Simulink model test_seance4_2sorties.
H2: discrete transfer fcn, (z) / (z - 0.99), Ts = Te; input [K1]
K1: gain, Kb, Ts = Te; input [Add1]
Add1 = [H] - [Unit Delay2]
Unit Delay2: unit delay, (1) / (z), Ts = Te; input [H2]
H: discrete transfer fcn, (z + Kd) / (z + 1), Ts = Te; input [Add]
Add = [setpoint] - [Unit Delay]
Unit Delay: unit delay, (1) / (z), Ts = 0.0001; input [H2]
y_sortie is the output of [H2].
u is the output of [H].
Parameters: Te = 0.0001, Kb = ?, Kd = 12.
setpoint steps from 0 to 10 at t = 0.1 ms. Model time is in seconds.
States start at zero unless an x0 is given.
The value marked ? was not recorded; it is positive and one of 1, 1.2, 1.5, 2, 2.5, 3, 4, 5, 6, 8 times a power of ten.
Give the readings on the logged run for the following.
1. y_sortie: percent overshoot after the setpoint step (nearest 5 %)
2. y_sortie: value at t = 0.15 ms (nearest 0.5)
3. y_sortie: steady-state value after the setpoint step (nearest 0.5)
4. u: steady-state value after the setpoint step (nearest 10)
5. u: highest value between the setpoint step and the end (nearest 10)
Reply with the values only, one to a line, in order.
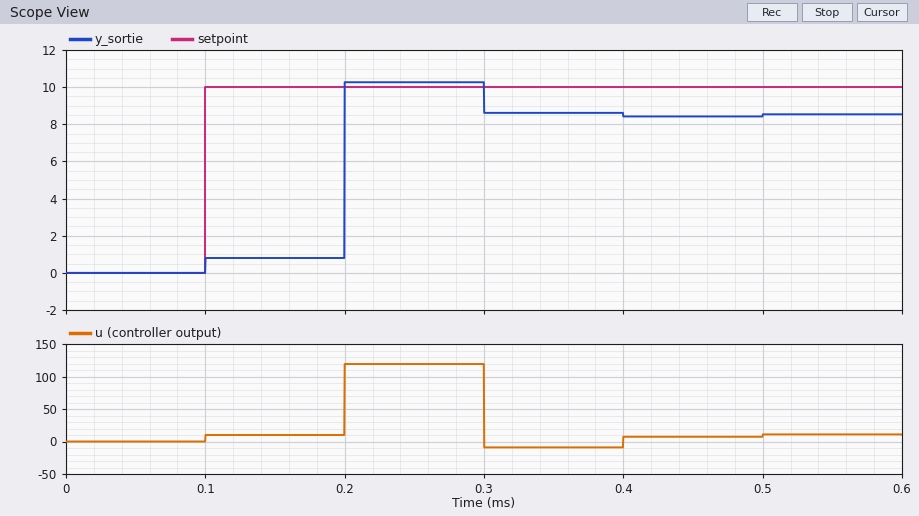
20 %
1.0
8.5
10
120
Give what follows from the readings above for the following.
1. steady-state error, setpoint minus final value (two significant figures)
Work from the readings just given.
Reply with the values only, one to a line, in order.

1.5
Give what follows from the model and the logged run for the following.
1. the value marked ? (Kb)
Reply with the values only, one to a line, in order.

0.08
